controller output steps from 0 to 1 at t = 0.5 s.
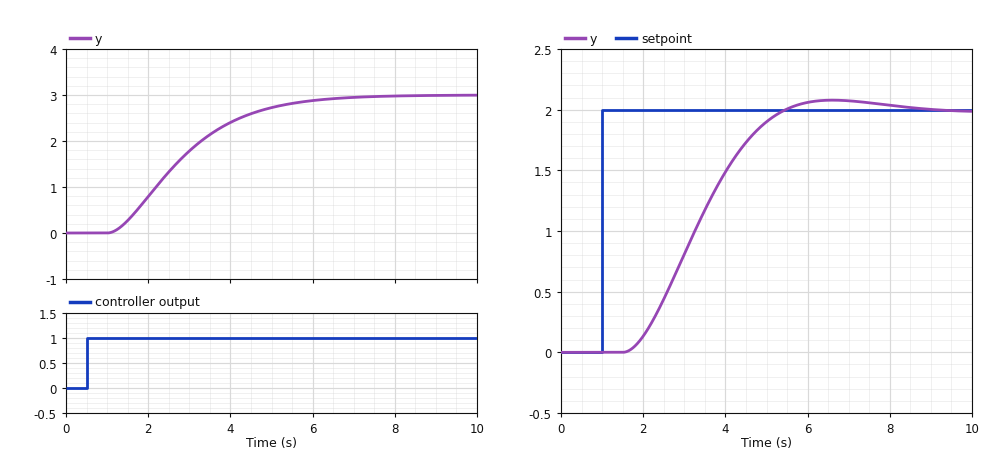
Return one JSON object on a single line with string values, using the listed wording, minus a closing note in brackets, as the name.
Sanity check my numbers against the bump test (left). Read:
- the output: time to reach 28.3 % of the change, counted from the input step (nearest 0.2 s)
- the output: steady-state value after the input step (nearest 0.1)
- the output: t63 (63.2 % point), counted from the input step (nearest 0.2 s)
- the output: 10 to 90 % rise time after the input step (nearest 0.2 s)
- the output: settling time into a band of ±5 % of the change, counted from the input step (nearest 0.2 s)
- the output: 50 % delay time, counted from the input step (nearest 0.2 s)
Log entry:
{"the output: time to reach 28.3 % of the change, counted from the input step": "1.6 s", "the output: steady-state value after the input step": "3.0", "the output: t63 (63.2 % point), counted from the input step": "2.6 s", "the output: 10 to 90 % rise time after the input step": "3.4 s", "the output: settling time into a band of ±5 % of the change, counted from the input step": "5.2 s", "the output: 50 % delay time, counted from the input step": "2.2 s"}
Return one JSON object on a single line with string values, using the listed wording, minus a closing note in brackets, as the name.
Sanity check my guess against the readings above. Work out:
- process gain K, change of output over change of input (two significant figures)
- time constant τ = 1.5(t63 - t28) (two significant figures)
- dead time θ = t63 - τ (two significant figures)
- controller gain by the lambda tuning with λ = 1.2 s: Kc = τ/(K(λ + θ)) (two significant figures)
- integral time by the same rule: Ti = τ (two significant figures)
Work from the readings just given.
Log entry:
{"process gain K, change of output over change of input": "3.0", "time constant τ = 1.5(t63 - t28)": "1.5 s", "dead time θ = t63 - τ": "1.1 s", "controller gain by the lambda tuning with λ = 1.2 s: Kc = τ/(K(λ + θ))": "0.22", "integral time by the same rule: Ti = τ": "1.5 s"}
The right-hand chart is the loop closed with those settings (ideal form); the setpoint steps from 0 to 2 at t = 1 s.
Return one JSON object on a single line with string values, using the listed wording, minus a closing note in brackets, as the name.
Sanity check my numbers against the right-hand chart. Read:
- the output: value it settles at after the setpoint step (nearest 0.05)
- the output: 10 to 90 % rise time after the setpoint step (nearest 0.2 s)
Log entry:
{"the output: value it settles at after the setpoint step": "2.00", "the output: 10 to 90 % rise time after the setpoint step": "2.6 s"}
